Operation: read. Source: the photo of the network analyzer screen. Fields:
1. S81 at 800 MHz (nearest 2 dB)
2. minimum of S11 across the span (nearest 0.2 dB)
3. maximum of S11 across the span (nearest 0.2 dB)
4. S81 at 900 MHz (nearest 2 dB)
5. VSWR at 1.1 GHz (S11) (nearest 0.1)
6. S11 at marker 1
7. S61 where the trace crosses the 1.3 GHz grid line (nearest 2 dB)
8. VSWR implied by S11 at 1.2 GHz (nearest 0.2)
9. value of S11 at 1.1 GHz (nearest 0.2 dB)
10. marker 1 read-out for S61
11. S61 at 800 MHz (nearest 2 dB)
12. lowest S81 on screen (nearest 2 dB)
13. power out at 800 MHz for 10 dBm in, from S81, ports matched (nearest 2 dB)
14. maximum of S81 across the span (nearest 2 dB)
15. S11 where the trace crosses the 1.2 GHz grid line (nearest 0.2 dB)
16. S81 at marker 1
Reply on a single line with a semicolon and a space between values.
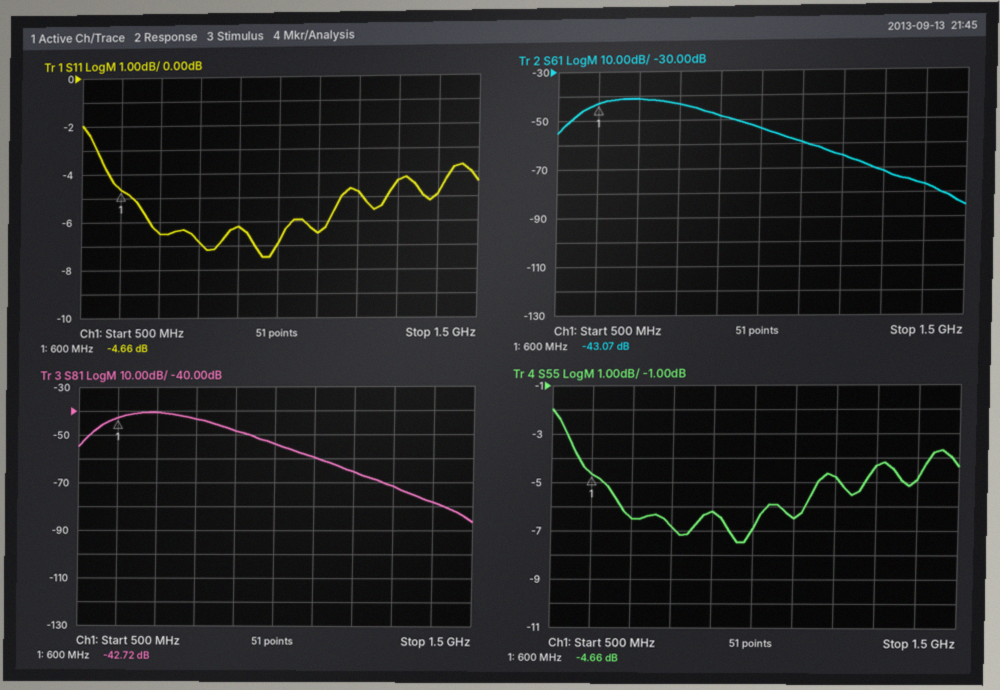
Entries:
-44 dB; -7.4 dB; -2.0 dB; -48 dB; 2.8; -4.66 dB; -72 dB; 3.8; -6.4 dB; -43.07 dB; -44 dB; -86 dB; -34 dBm; -40 dB; -4.8 dB; -42.72 dB
